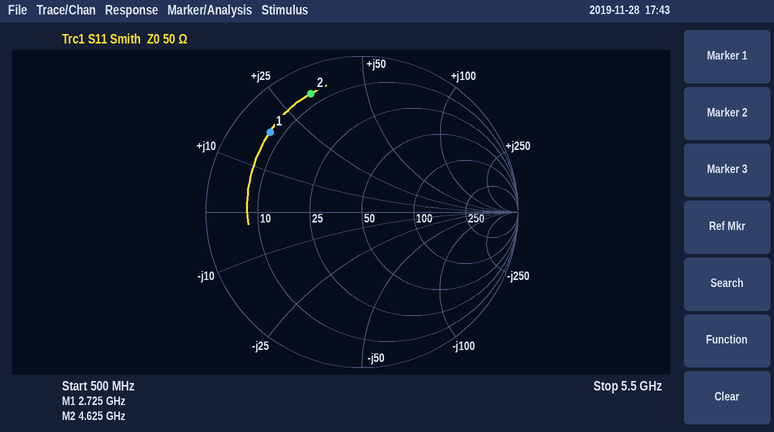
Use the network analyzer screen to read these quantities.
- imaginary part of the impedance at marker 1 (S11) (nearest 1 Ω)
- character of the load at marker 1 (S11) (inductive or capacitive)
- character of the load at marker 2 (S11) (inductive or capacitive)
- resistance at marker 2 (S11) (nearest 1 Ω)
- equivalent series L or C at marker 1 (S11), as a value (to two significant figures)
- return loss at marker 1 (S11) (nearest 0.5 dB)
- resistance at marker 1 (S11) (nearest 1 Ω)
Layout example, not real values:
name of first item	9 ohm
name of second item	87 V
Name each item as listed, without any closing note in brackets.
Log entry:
imaginary part of the impedance at marker 1 (S11)	+18 Ω
character of the load at marker 1 (S11)	inductive
character of the load at marker 2 (S11)	inductive
resistance at marker 2 (S11)	7 Ω
equivalent series L or C at marker 1 (S11), as a value	1.1 nH
return loss at marker 1 (S11)	2.0 dB
resistance at marker 1 (S11)	7 Ω
